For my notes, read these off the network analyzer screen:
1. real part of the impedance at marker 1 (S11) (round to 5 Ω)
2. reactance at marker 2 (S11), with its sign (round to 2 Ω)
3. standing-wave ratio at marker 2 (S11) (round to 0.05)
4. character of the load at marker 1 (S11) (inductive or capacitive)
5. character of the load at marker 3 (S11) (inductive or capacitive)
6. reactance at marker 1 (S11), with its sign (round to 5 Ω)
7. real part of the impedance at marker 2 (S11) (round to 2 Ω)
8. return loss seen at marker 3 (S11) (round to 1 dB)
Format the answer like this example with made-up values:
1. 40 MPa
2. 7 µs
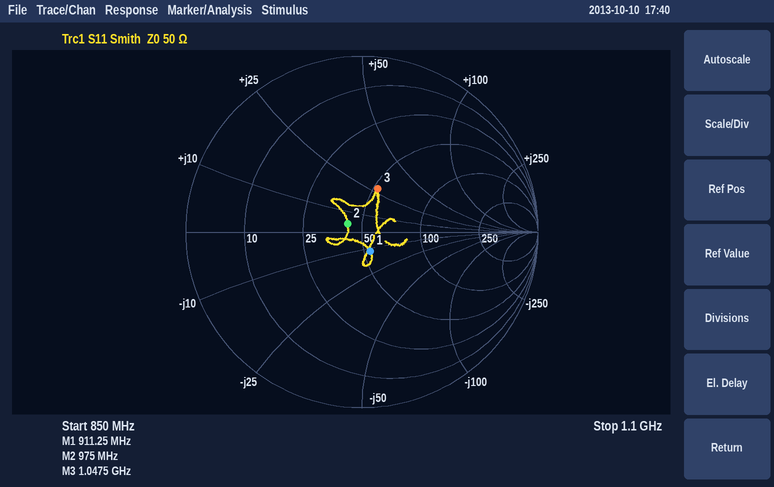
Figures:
1. 55 Ω
2. +4 Ω
3. 1.20
4. capacitive
5. inductive
6. -10 Ω
7. 42 Ω
8. 12 dB
